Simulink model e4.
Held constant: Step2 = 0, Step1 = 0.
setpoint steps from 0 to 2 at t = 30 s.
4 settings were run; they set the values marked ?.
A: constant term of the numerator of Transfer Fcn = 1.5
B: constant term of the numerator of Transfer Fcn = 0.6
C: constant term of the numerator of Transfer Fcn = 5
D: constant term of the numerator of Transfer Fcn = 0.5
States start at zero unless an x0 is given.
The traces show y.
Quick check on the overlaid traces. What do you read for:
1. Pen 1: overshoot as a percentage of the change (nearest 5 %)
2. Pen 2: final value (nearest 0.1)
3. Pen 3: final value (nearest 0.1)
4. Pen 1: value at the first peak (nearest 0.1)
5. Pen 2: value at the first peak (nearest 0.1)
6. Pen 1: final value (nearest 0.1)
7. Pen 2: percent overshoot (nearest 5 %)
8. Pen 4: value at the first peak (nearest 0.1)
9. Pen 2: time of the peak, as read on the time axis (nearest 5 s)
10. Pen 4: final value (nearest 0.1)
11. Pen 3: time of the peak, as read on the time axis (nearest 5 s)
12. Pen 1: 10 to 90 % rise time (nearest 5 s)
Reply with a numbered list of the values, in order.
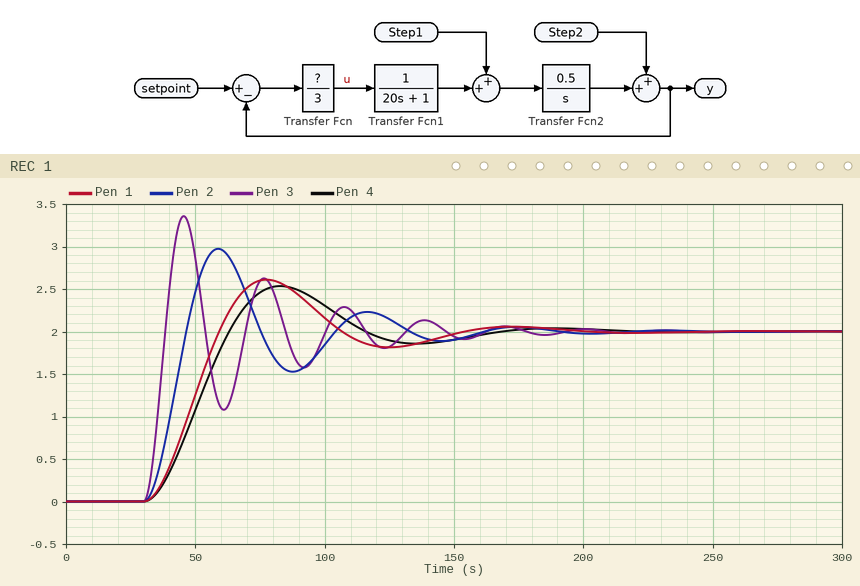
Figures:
1. 30 %
2. 2.0
3. 2.0
4. 2.6
5. 3.0
6. 2.0
7. 50 %
8. 2.5
9. 60 s
10. 2.0
11. 45 s
12. 20 s
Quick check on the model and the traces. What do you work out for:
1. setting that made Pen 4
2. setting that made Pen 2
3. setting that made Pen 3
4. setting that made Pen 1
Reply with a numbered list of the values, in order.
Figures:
1. D
2. A
3. C
4. B
